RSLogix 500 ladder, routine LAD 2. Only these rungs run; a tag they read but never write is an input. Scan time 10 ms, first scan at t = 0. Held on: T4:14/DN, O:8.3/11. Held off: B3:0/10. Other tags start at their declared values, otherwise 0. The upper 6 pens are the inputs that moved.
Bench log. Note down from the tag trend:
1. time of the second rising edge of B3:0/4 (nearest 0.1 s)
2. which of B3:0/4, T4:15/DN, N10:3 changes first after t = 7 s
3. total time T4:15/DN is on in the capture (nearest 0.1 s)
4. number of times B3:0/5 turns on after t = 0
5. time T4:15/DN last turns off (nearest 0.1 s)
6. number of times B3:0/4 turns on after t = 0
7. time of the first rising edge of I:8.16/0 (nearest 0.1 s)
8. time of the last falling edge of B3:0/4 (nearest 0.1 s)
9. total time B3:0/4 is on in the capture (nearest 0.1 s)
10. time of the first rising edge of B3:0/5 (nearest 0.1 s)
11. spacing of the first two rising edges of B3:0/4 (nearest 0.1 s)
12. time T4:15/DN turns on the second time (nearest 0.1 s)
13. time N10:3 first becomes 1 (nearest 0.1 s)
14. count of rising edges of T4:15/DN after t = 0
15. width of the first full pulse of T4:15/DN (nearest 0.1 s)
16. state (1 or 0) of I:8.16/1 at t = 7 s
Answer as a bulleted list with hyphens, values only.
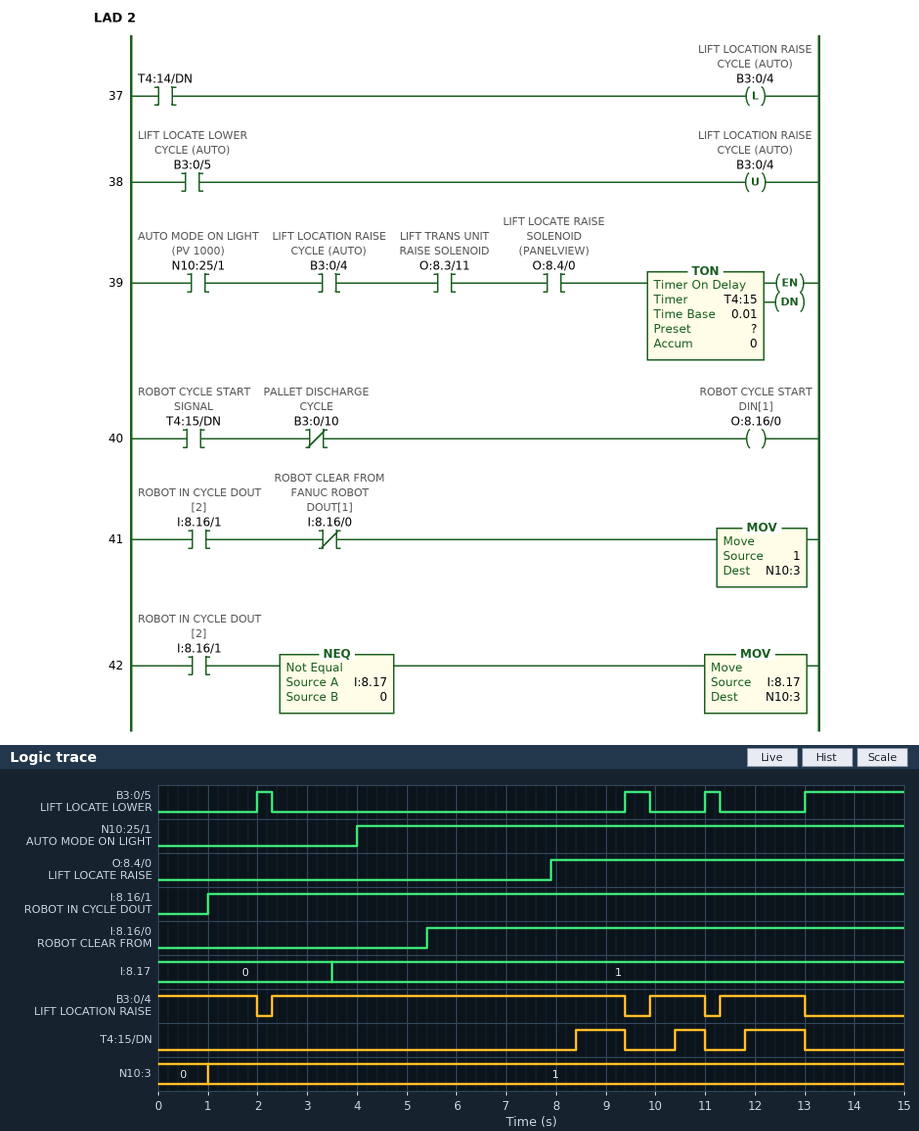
- 9.9 s
- T4:15/DN
- 2.8 s
- 4
- 13.0 s
- 3
- 5.4 s
- 13.0 s
- 11.9 s
- 2.0 s
- 7.6 s
- 10.4 s
- 1.0 s
- 3
- 1.0 s
- 1
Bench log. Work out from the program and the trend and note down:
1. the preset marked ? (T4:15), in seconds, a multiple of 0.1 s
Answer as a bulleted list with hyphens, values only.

- 0.5 s
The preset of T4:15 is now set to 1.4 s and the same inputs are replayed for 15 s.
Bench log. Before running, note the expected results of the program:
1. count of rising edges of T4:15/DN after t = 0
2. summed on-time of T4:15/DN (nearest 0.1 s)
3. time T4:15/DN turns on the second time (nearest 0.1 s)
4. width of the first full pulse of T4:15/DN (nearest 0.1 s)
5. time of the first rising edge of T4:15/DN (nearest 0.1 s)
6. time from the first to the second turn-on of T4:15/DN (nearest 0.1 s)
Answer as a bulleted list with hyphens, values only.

- 2
- 0.4 s
- 12.7 s
- 0.1 s
- 9.3 s
- 3.4 s
